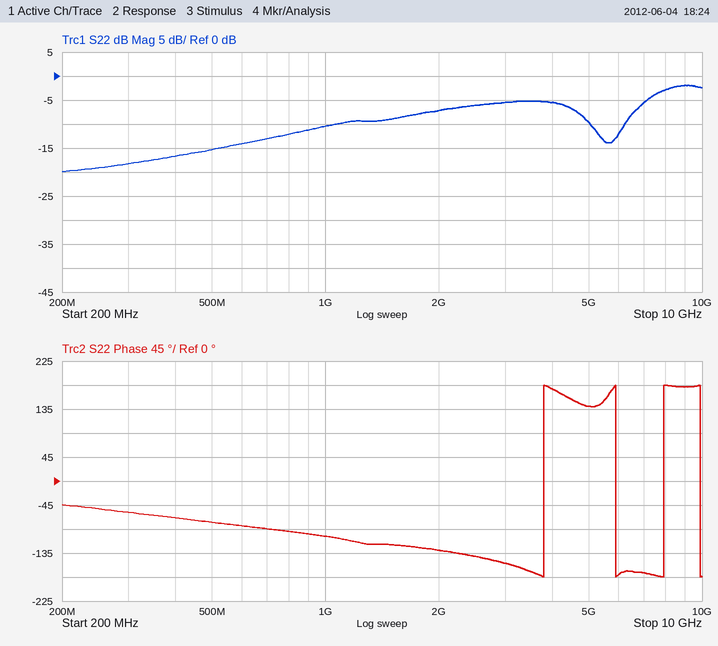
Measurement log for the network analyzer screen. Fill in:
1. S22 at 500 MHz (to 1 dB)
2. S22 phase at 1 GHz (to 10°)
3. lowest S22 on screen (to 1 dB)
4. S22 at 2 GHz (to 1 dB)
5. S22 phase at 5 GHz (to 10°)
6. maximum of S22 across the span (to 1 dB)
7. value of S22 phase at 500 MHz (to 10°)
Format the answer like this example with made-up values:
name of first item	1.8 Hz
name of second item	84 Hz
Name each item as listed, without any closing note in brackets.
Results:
S22 at 500 MHz	-15 dB
S22 phase at 1 GHz	-100°
lowest S22 on screen	-20 dB
S22 at 2 GHz	-7 dB
S22 phase at 5 GHz	140°
maximum of S22 across the span	-2 dB
value of S22 phase at 500 MHz	-80°
